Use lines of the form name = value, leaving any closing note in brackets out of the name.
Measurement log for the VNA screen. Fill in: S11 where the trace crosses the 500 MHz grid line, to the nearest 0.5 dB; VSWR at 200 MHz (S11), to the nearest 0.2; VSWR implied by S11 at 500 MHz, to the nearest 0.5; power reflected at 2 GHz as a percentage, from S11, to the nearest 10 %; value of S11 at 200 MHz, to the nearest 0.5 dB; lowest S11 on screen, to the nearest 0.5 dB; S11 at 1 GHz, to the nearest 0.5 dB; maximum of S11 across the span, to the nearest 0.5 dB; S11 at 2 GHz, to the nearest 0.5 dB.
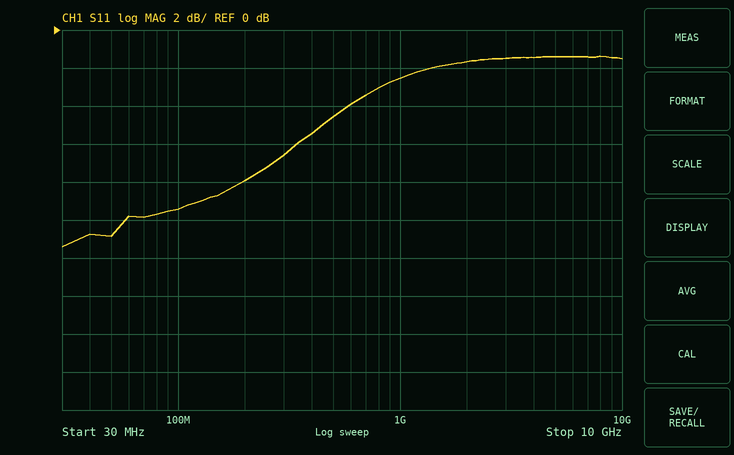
S11 where the trace crosses the 500 MHz grid line, to the nearest 0.5 dB = -4.5 dB
VSWR at 200 MHz (S11), to the nearest 0.2 = 2.4
VSWR implied by S11 at 500 MHz, to the nearest 0.5 = 4.0
power reflected at 2 GHz as a percentage, from S11, to the nearest 10 % = 70 %
value of S11 at 200 MHz, to the nearest 0.5 dB = -8.0 dB
lowest S11 on screen, to the nearest 0.5 dB = -11.5 dB
S11 at 1 GHz, to the nearest 0.5 dB = -2.5 dB
maximum of S11 across the span, to the nearest 0.5 dB = -1.5 dB
S11 at 2 GHz, to the nearest 0.5 dB = -1.5 dB
